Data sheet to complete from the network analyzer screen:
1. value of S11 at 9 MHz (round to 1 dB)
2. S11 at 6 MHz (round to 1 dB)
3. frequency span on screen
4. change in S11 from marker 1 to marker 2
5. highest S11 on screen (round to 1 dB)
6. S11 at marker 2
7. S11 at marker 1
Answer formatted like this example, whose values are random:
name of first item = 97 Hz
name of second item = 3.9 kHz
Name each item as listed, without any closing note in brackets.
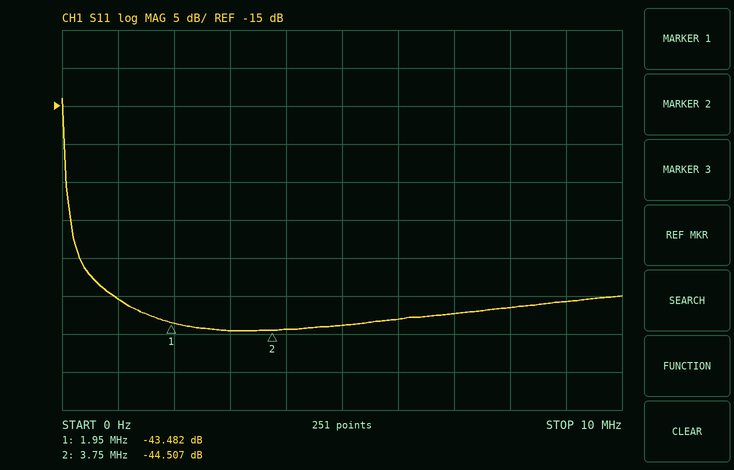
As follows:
value of S11 at 9 MHz = -41 dB
S11 at 6 MHz = -43 dB
frequency span on screen = 10 MHz
change in S11 from marker 1 to marker 2 = -1.025 dB
highest S11 on screen = -14 dB
S11 at marker 2 = -44.507 dB
S11 at marker 1 = -43.482 dB
